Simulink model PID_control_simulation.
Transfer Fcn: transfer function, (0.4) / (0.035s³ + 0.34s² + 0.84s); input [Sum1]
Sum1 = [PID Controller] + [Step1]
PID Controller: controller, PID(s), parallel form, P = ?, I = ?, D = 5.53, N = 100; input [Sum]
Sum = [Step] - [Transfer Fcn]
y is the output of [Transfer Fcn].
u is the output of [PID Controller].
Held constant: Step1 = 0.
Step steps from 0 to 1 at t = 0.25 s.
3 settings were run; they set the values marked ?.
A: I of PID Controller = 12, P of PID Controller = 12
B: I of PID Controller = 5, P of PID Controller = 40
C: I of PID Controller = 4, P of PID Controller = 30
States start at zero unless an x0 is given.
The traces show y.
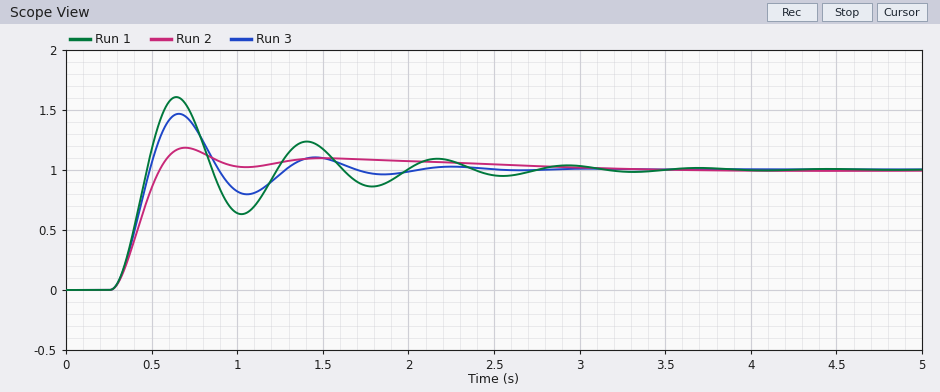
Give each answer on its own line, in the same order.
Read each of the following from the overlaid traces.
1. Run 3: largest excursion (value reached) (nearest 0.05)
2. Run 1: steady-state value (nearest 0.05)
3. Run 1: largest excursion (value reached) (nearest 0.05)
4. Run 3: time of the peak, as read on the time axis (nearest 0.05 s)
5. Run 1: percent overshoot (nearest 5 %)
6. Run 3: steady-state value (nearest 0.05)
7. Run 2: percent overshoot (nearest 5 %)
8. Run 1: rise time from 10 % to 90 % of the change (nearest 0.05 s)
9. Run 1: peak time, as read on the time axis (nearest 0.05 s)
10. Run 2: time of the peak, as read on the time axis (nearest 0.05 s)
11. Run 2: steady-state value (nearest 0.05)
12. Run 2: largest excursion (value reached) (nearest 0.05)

1.45
1.00
1.60
0.65 s
60 %
1.00
20 %
0.15 s
0.65 s
0.70 s
1.00
1.20
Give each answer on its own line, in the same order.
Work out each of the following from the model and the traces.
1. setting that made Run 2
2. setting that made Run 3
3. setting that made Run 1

A
C
B
